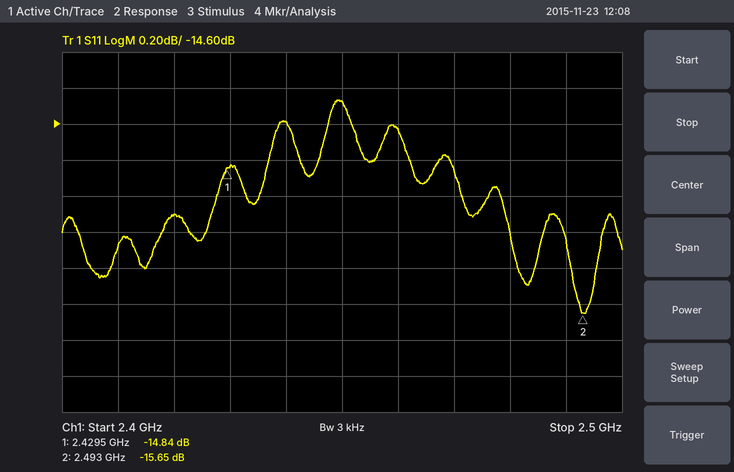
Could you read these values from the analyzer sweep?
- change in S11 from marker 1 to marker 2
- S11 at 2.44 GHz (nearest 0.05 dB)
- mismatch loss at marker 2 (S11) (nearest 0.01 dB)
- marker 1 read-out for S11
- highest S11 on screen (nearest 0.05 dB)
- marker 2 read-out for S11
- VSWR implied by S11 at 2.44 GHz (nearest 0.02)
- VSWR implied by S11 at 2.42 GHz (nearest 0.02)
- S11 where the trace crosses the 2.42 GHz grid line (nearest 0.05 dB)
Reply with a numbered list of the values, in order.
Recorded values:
1. -0.81 dB
2. -14.60 dB
3. 0.12 dB
4. -14.84 dB
5. -14.45 dB
6. -15.65 dB
7. 1.46
8. 1.42
9. -15.10 dB
